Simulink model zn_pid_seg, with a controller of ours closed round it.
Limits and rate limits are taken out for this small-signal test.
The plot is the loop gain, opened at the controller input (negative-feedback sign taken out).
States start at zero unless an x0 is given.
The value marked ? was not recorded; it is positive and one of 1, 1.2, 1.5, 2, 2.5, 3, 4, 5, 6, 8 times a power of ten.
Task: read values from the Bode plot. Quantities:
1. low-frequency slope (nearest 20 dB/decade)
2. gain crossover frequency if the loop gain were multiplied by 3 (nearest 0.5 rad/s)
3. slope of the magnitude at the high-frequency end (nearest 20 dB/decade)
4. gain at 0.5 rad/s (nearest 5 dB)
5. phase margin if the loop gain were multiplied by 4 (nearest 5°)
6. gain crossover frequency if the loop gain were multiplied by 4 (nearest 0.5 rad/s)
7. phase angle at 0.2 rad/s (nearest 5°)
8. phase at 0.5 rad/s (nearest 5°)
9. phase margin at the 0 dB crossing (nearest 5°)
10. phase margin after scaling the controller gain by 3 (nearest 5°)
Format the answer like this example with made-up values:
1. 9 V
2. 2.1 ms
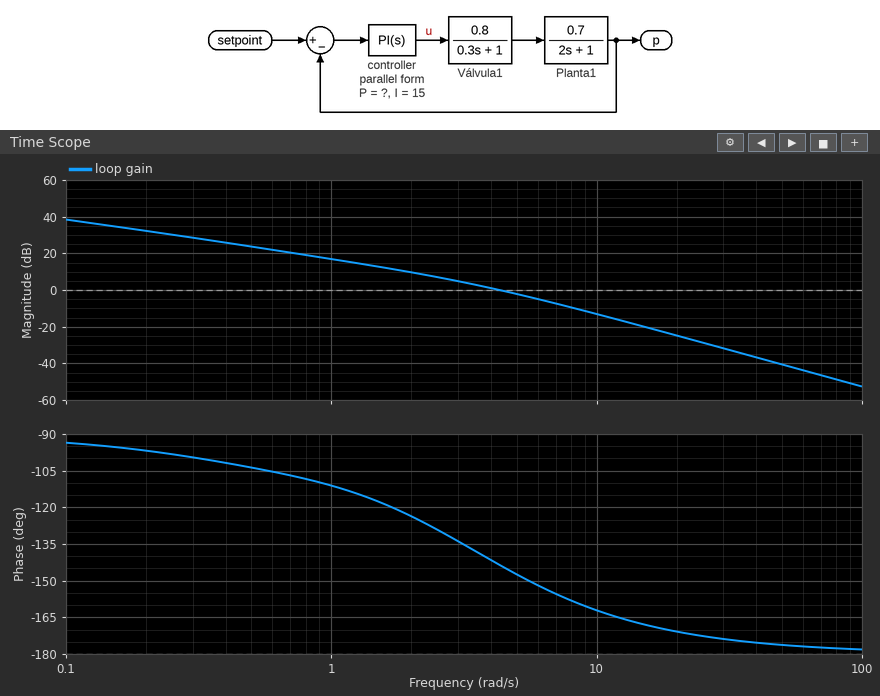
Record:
1. -20 dB/decade
2. 8.0 rad/s
3. -40 dB/decade
4. 25 dB
5. 20°
6. 9.5 rad/s
7. -95°
8. -105°
9. 35°
10. 20°
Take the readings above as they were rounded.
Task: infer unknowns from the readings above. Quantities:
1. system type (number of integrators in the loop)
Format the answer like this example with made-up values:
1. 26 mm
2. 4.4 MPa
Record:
1. 1
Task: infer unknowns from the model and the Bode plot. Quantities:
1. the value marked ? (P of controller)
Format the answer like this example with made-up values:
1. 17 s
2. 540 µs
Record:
1. 25
